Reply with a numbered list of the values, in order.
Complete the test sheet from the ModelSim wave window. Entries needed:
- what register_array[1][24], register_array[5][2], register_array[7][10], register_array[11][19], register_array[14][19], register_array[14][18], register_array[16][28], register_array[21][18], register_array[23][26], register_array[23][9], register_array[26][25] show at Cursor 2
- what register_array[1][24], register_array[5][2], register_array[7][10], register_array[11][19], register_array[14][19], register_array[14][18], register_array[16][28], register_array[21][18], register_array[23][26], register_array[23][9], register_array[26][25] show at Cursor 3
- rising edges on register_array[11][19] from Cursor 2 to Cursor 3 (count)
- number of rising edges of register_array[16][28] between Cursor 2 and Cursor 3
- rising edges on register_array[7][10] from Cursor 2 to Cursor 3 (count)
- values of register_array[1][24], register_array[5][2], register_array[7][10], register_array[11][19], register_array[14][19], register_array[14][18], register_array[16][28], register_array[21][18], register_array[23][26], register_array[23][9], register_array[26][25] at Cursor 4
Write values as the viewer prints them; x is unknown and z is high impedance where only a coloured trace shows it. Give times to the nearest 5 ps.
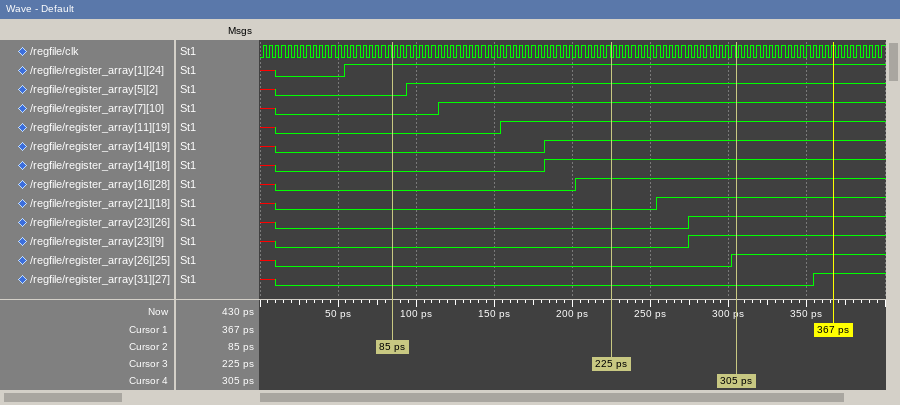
1. register_array[1][24]=1, register_array[5][2]=0, register_array[7][10]=0, register_array[11][19]=0, register_array[14][19]=0, register_array[14][18]=0, register_array[16][28]=0, register_array[21][18]=0, register_array[23][26]=0, register_array[23][9]=0, register_array[26][25]=0
2. register_array[1][24]=1, register_array[5][2]=1, register_array[7][10]=1, register_array[11][19]=1, register_array[14][19]=1, register_array[14][18]=1, register_array[16][28]=1, register_array[21][18]=0, register_array[23][26]=0, register_array[23][9]=0, register_array[26][25]=0
3. 1
4. 1
5. 1
6. register_array[1][24]=1, register_array[5][2]=1, register_array[7][10]=1, register_array[11][19]=1, register_array[14][19]=1, register_array[14][18]=1, register_array[16][28]=1, register_array[21][18]=1, register_array[23][26]=1, register_array[23][9]=1, register_array[26][25]=1
